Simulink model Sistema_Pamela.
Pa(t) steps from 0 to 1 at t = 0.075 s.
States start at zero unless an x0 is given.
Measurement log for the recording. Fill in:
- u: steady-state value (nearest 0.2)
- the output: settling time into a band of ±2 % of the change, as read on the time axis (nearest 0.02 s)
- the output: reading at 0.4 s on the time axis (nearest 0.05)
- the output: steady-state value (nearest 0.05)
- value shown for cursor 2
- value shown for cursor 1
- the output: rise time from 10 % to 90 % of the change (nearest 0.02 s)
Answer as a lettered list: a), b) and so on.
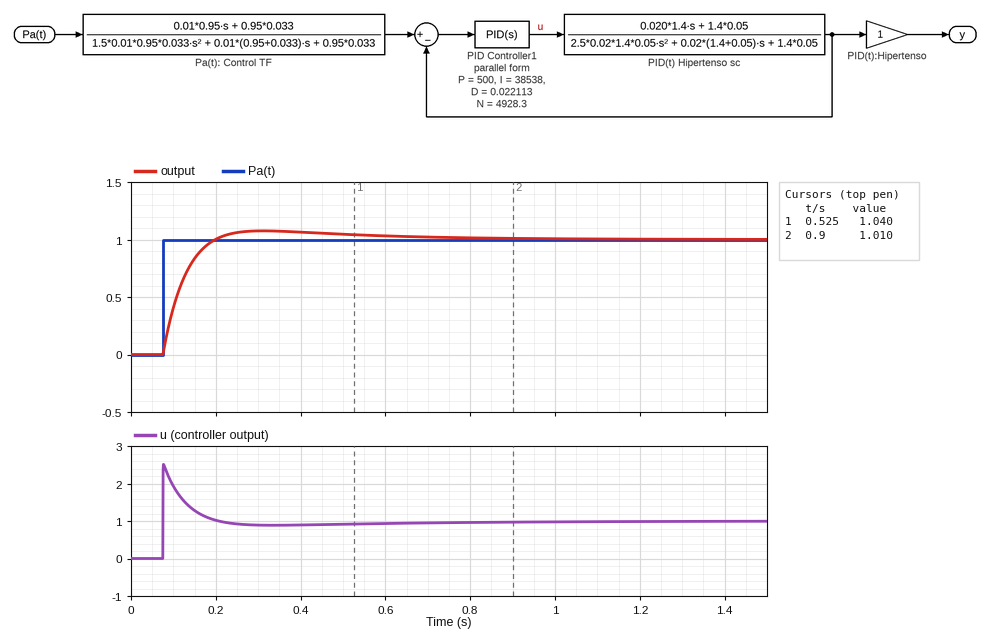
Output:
a) 1.0
b) 0.72 s
c) 1.05
d) 1.00
e) 1.010
f) 1.040
g) 0.08 s
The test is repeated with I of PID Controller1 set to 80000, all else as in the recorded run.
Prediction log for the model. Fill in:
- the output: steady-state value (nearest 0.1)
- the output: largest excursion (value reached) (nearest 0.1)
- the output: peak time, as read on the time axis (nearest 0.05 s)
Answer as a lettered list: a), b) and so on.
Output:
a) 1.0
b) 1.1
c) 0.30 s
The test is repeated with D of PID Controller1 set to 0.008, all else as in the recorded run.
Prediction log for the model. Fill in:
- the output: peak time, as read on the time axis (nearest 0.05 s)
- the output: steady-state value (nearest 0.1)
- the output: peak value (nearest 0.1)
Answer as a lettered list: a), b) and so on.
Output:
a) 0.30 s
b) 1.0
c) 1.1
